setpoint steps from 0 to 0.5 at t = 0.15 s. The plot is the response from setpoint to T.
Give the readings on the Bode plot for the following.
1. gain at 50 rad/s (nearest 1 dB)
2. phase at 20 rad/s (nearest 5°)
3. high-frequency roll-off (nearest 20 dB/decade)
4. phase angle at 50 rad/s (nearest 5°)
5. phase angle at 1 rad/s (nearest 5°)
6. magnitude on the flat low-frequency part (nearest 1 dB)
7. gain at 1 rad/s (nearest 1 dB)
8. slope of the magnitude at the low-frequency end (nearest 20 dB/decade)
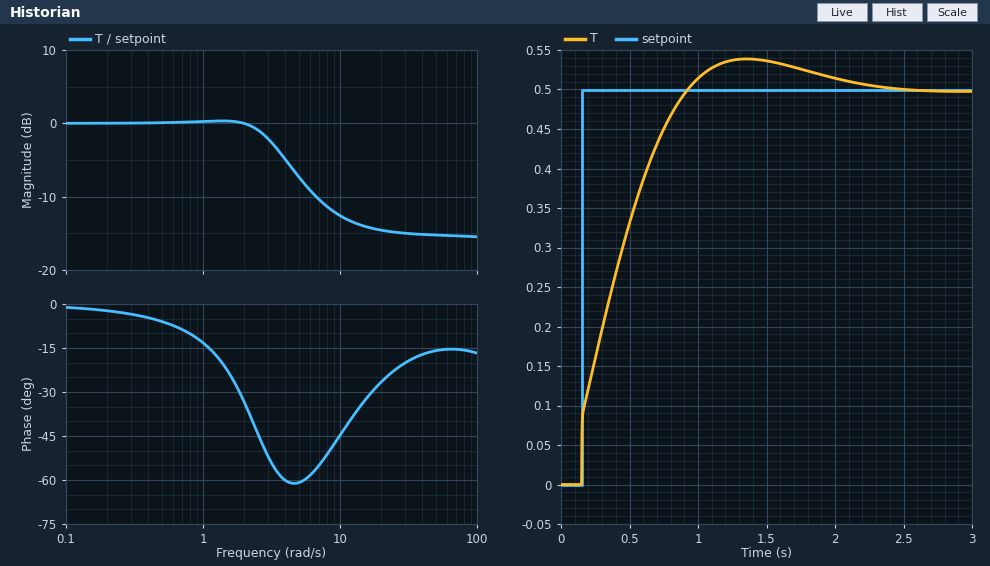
-15 dB
-25°
0 dB/decade
-15°
-15°
0 dB
0 dB
0 dB/decade
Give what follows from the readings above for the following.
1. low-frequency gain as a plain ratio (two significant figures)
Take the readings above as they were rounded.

1.0
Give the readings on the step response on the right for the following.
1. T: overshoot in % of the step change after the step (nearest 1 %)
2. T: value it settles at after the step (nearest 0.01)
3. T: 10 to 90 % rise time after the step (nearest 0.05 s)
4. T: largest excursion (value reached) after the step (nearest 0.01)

8 %
0.50
0.60 s
0.54
